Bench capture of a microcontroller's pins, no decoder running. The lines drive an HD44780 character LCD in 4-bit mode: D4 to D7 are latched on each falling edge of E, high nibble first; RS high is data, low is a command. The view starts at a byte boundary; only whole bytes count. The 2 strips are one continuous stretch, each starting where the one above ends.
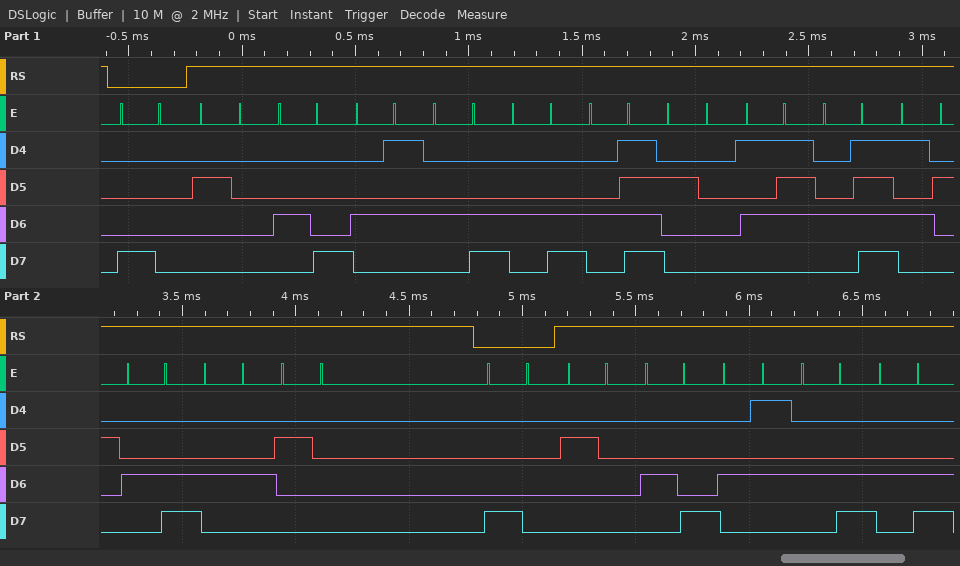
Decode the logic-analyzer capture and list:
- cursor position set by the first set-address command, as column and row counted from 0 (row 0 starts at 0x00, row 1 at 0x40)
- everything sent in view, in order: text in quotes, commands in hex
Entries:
column 0, row 0
0x80 " HELLO WORLD " 0x80 " HELL"
